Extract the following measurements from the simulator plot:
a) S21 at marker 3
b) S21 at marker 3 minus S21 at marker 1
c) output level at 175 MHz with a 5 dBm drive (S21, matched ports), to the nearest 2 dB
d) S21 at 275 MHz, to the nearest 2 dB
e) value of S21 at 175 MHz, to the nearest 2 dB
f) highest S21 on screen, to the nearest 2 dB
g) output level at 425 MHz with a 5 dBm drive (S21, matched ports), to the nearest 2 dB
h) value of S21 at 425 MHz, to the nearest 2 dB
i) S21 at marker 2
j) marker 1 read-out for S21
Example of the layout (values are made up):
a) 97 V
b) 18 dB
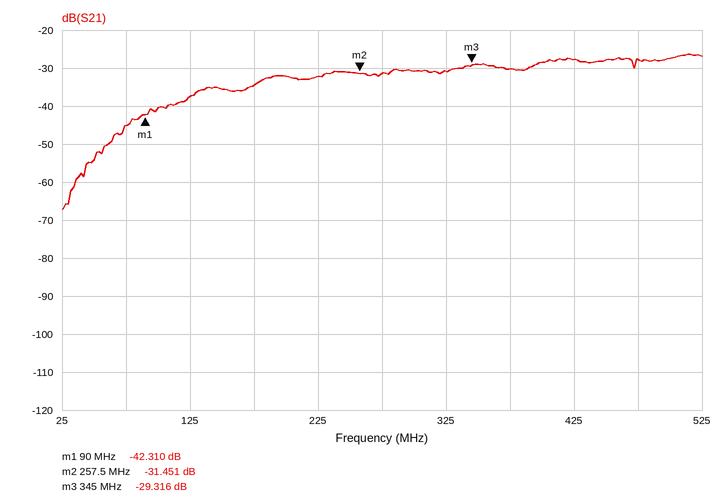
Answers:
a) -29.316 dB
b) 12.994 dB
c) -30 dBm
d) -32 dB
e) -34 dB
f) -26 dB
g) -22 dBm
h) -28 dB
i) -31.451 dB
j) -42.310 dB
